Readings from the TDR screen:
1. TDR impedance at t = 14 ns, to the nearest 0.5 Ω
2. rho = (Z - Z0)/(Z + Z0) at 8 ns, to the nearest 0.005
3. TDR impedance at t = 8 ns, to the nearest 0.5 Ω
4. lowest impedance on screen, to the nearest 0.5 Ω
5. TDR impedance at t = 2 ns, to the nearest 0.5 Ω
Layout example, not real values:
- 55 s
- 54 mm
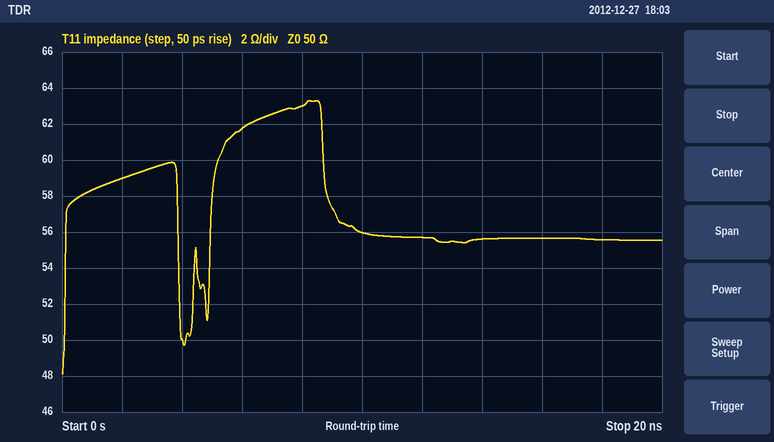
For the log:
- 55.5 Ω
- +0.115
- 63.0 Ω
- 48.0 Ω
- 59.0 Ω
